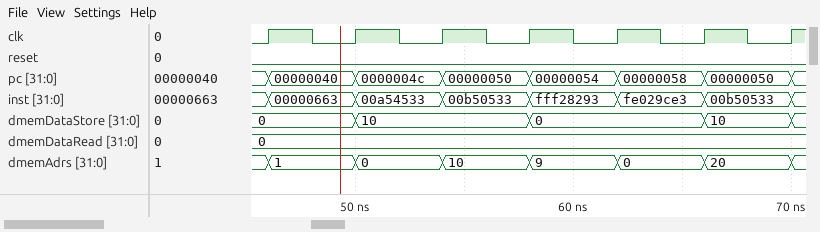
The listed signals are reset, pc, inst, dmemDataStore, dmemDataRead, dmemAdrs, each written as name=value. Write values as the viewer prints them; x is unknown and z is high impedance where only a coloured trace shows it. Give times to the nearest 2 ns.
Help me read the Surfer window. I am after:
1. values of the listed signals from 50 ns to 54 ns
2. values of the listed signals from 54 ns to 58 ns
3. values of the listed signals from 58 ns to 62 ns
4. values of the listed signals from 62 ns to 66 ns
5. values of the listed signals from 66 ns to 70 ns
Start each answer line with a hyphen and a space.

- reset=0, pc=0000004c, inst=00a54533, dmemDataStore=10, dmemDataRead=0, dmemAdrs=0
- reset=0, pc=00000050, inst=00b50533, dmemDataStore=10, dmemDataRead=0, dmemAdrs=10
- reset=0, pc=00000054, inst=fff28293, dmemDataStore=0, dmemDataRead=0, dmemAdrs=9
- reset=0, pc=00000058, inst=fe029ce3, dmemDataStore=0, dmemDataRead=0, dmemAdrs=0
- reset=0, pc=00000050, inst=00b50533, dmemDataStore=10, dmemDataRead=0, dmemAdrs=20
